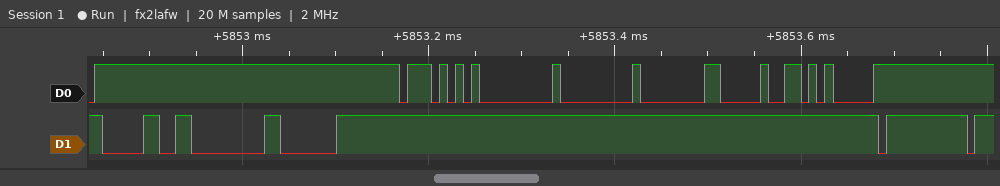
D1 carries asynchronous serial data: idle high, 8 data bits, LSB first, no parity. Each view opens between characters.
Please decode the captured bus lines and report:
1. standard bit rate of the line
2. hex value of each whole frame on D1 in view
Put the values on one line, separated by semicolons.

115200 baud; 30, 00, C0, FF
